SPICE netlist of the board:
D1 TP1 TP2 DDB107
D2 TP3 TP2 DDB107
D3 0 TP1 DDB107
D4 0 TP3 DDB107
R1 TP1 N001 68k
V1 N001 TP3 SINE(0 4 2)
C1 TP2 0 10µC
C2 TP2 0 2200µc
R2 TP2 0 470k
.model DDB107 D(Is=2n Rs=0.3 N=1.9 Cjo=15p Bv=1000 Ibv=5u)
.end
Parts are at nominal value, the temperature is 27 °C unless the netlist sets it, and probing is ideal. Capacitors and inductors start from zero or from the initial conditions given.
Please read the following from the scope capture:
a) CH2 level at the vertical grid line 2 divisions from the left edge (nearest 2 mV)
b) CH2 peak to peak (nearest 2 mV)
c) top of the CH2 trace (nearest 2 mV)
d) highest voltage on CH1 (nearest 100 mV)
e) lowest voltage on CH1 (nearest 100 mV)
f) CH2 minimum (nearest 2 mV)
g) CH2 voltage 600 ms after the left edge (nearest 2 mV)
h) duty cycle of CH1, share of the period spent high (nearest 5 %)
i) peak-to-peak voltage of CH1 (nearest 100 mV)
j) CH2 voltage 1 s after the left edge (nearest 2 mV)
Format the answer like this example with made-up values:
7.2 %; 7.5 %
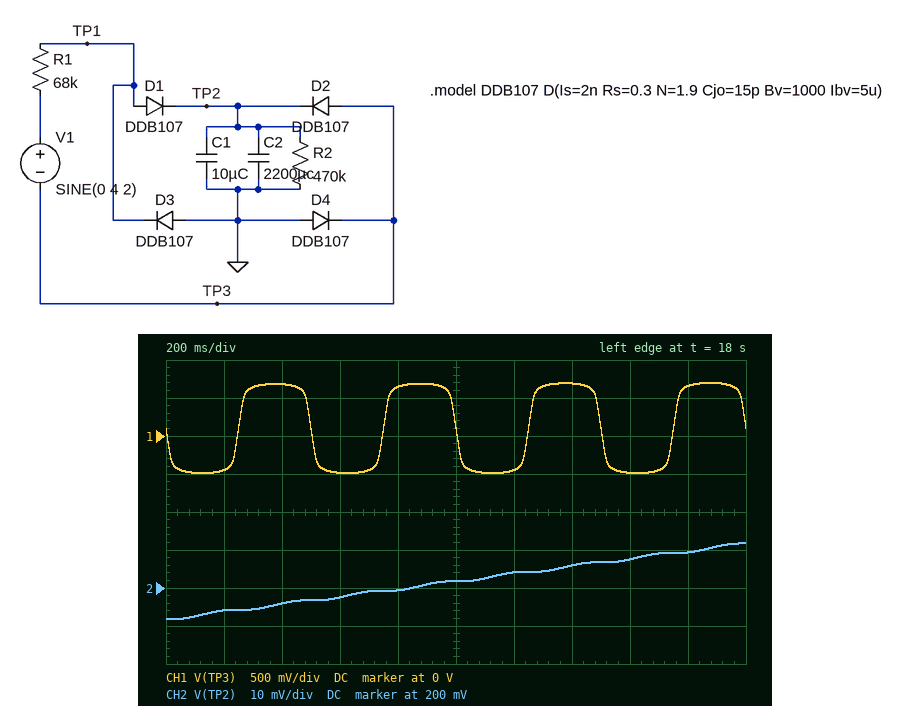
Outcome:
196 mV; 20 mV; 212 mV; 700 mV; -500 mV; 192 mV; 198 mV; 50 %; 1.2 V; 202 mV
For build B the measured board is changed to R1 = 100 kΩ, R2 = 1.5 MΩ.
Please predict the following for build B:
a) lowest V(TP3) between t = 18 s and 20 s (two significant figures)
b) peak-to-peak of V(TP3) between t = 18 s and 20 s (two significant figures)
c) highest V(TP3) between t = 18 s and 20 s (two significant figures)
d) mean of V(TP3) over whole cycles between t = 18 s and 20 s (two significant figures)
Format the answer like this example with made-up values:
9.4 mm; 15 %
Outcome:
-470 mV; 1.1 V; 620 mV; 72 mV
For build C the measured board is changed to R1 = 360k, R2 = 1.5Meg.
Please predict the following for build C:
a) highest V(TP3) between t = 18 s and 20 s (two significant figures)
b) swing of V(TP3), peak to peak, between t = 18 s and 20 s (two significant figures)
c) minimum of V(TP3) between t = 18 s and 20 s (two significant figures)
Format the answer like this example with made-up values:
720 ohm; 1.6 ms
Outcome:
460 mV; 870 mV; -410 mV
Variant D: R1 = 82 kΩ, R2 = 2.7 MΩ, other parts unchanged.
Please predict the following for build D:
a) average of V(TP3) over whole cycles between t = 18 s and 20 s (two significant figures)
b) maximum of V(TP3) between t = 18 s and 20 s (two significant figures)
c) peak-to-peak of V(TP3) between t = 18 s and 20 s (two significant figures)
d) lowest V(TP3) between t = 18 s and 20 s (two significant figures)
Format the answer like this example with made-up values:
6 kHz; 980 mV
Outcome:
86 mV; 660 mV; 1.1 V; -480 mV
